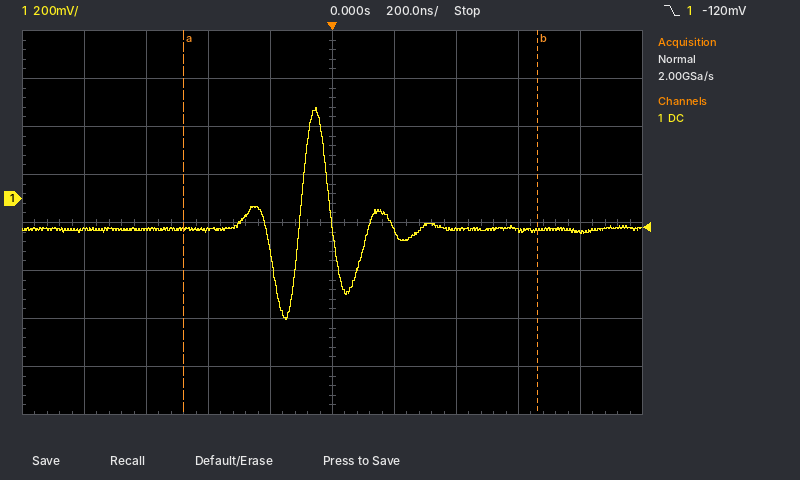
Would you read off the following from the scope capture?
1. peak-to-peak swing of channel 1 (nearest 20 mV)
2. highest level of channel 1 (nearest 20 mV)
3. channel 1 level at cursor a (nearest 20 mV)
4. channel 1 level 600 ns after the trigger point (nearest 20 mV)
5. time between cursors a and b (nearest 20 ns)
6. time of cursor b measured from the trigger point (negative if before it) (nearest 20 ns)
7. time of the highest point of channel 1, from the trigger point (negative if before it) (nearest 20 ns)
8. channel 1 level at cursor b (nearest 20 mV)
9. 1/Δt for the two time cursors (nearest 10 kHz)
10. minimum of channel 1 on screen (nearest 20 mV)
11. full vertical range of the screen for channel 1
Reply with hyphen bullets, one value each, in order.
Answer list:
- 880 mV
- 380 mV
- -120 mV
- -140 mV
- 1.14 µs
- +660 ns
- -60 ns
- -140 mV
- 880 kHz
- -500 mV
- 1.6 V
